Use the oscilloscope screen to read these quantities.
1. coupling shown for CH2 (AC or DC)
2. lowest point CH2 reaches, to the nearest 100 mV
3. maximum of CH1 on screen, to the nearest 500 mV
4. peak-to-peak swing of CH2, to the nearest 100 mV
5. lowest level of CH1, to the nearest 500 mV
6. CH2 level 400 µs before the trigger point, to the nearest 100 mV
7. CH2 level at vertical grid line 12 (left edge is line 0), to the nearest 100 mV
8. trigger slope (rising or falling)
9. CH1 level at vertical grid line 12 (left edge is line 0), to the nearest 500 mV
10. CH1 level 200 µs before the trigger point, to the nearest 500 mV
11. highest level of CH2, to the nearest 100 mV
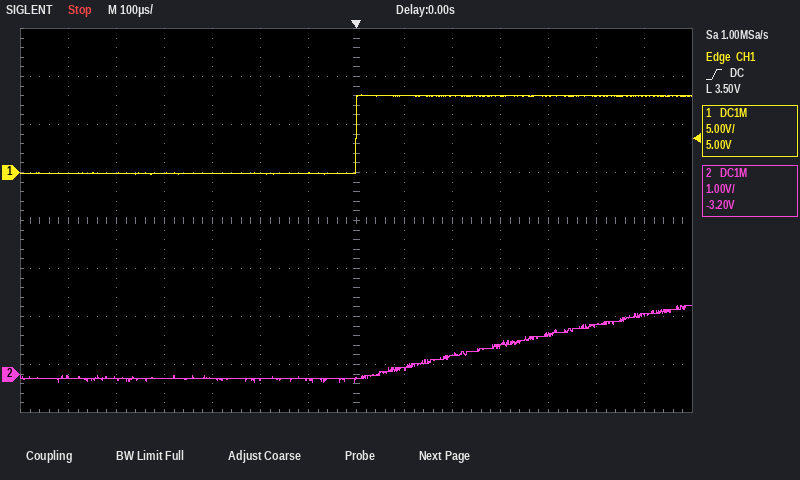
DC
-200 mV
8.0 V
1.6 V
0.0 V
-100 mV
1.0 V
rising
8.0 V
0.0 V
1.4 V
